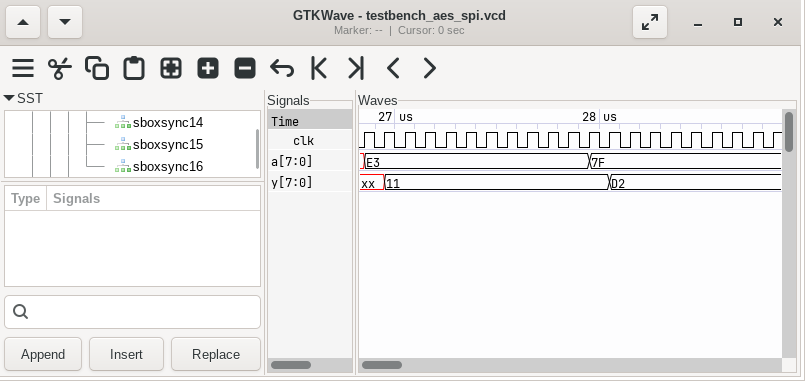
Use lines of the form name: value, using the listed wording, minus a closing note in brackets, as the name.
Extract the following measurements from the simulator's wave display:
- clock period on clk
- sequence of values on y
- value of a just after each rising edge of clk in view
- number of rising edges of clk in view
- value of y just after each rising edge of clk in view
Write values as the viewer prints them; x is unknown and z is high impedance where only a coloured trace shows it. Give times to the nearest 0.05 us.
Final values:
clock period on clk: 0.1 us
sequence of values on y: xx, 11, D2
value of a just after each rising edge of clk in view: E3, E3, E3, E3, E3, E3, E3, E3, E3, E3, E3, 7F, 7F, 7F, 7F, 7F, 7F, 7F, 7F, 7F, 7F
number of rising edges of clk in view: 21
value of y just after each rising edge of clk in view: xx, 11, 11, 11, 11, 11, 11, 11, 11, 11, 11, 11, D2, D2, D2, D2, D2, D2, D2, D2, D2
